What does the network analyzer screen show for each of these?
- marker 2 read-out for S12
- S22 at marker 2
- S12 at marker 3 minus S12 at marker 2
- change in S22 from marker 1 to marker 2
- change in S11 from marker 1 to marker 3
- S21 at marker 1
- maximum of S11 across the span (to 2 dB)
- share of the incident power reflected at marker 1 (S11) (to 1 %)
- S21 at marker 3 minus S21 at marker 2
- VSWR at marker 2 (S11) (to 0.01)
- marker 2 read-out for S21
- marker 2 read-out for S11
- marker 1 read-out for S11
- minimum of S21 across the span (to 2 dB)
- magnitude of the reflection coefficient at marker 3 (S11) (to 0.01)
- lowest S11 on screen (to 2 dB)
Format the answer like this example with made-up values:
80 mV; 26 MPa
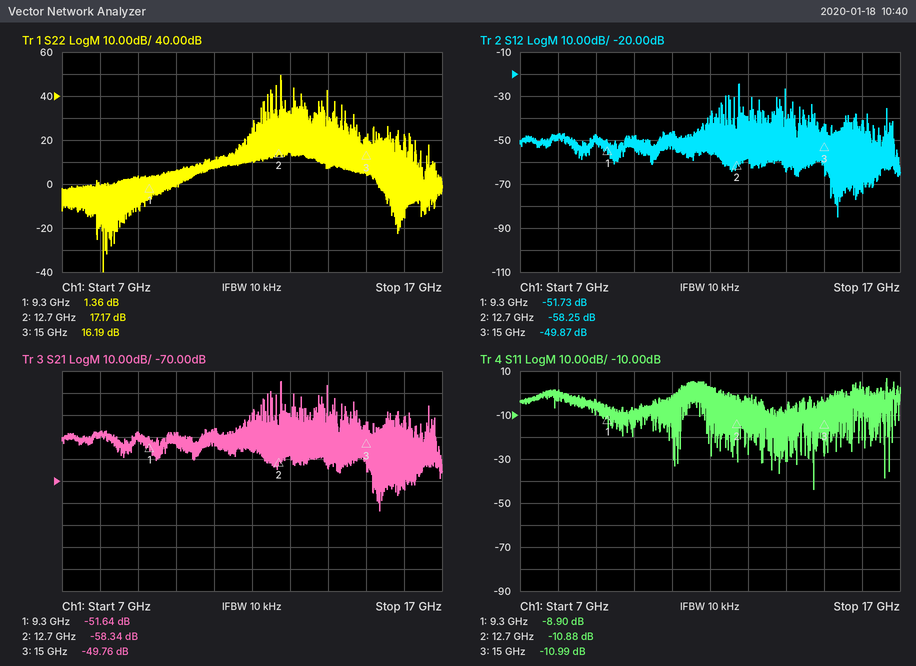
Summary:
-58.25 dB; 17.17 dB; 8.38 dB; 15.81 dB; -2.09 dB; -51.64 dB; 6 dB; 13 %; 8.58 dB; 1.80; -58.34 dB; -10.88 dB; -8.90 dB; -84 dB; 0.28; -44 dB
